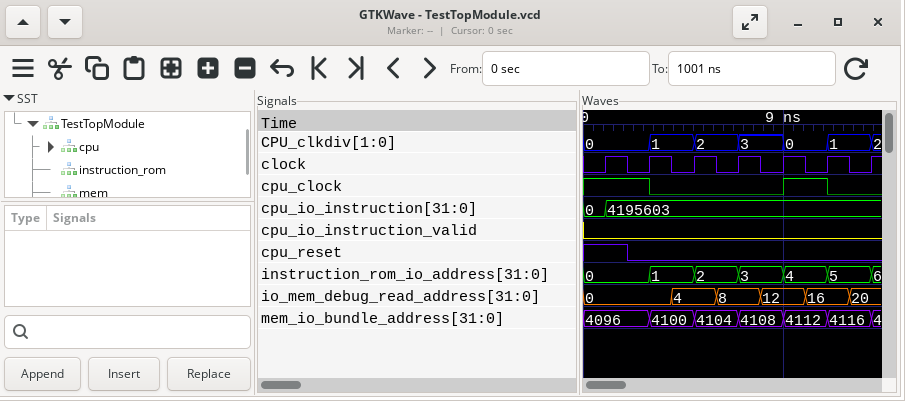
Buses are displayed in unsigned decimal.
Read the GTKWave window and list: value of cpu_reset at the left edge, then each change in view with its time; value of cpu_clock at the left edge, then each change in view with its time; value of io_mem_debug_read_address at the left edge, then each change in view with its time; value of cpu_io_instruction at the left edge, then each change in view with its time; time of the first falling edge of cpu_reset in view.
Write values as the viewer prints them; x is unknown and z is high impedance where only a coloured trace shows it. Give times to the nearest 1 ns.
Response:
1, 0 at 2 ns
1, 0 at 3 ns, 1 at 9 ns, 0 at 11 ns
0, 4 at 4 ns, 8 at 6 ns, 12 at 8 ns, 16 at 10 ns, 20 at 12 ns
0, 4195603 at 1 ns
2 ns
